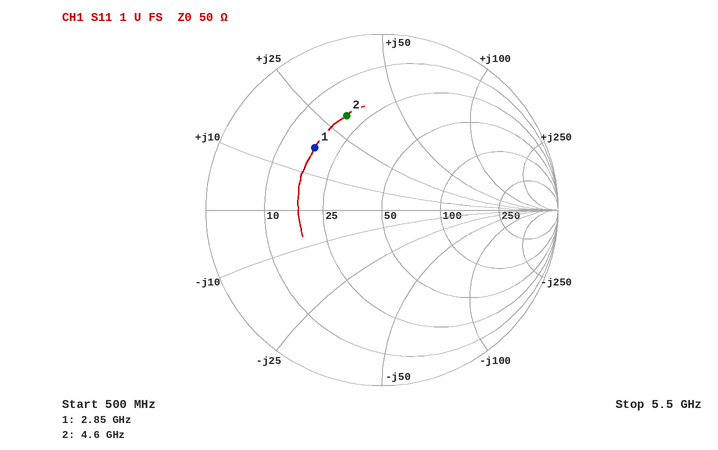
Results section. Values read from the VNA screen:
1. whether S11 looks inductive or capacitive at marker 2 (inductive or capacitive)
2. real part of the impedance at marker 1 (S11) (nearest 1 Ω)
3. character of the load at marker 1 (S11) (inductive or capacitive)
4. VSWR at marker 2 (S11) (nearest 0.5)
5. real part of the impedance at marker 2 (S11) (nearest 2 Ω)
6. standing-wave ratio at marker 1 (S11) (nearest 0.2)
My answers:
inductive
18 Ω
inductive
3.5
20 Ω
3.2
